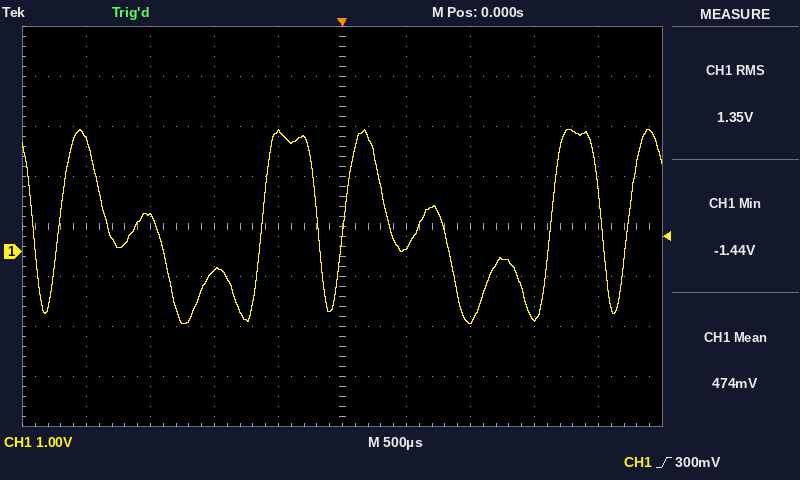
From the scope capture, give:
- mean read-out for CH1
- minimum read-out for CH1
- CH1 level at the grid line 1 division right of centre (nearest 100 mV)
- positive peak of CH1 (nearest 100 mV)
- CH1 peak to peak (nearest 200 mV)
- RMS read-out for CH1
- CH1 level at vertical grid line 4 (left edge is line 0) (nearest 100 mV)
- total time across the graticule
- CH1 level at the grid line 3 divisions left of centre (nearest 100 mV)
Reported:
474 mV
-1.44 V
100 mV
2.4 V
3.8 V
1.35 V
2.4 V
5 ms
700 mV
